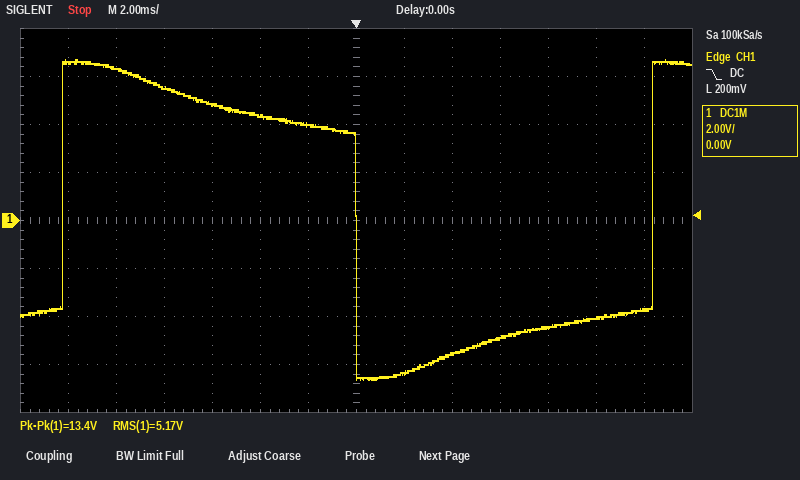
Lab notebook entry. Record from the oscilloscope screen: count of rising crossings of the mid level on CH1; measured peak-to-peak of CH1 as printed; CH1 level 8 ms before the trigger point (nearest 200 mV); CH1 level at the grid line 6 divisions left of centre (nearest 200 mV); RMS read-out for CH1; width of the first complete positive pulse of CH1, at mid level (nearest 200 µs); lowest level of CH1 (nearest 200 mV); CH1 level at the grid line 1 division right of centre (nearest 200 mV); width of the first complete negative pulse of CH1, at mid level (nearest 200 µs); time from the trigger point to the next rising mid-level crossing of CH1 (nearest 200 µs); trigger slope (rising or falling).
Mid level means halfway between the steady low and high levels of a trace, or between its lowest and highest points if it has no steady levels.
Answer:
2
13.4 V
5.6 V
6.6 V
5.17 V
12.2 ms
-6.6 V
-6.4 V
12.4 ms
12.4 ms
falling
